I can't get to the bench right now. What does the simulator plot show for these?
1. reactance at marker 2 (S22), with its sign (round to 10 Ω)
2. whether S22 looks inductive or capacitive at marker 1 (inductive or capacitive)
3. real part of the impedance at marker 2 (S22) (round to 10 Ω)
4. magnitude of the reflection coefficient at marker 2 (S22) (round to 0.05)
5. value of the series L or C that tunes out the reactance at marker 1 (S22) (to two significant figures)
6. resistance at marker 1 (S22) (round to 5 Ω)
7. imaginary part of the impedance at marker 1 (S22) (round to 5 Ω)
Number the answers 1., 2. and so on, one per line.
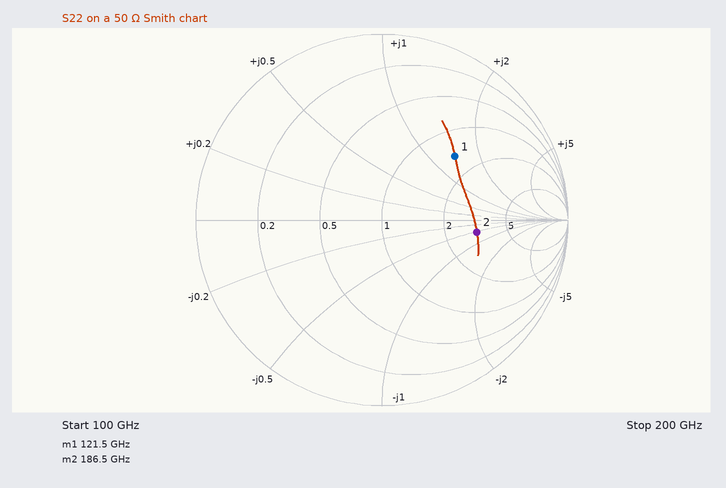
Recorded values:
1. -30 Ω
2. inductive
3. 150 Ω
4. 0.50
5. 19 fF
6. 75 Ω
7. +70 Ω
